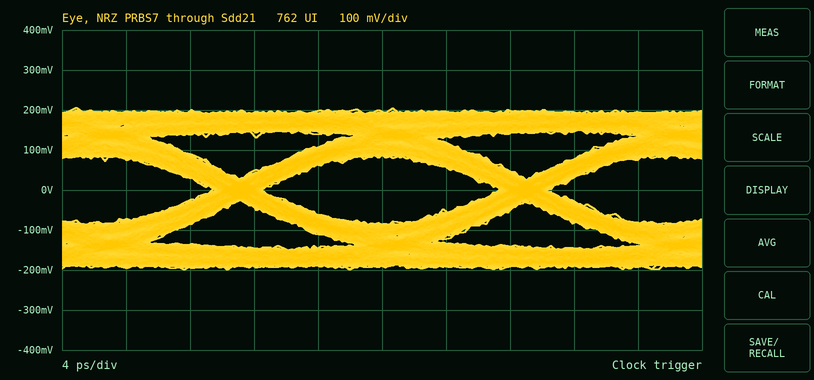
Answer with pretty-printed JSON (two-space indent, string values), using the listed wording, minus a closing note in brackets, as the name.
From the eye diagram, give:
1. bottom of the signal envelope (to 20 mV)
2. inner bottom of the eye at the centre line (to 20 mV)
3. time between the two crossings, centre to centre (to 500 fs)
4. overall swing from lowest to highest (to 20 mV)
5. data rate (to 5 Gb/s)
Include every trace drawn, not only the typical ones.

{
  "bottom of the signal envelope": "-200 mV",
  "inner bottom of the eye at the centre line": "-80 mV",
  "time between the two crossings, centre to centre": "18.0 ps",
  "overall swing from lowest to highest": "400 mV",
  "data rate": "55 Gb/s"
}
